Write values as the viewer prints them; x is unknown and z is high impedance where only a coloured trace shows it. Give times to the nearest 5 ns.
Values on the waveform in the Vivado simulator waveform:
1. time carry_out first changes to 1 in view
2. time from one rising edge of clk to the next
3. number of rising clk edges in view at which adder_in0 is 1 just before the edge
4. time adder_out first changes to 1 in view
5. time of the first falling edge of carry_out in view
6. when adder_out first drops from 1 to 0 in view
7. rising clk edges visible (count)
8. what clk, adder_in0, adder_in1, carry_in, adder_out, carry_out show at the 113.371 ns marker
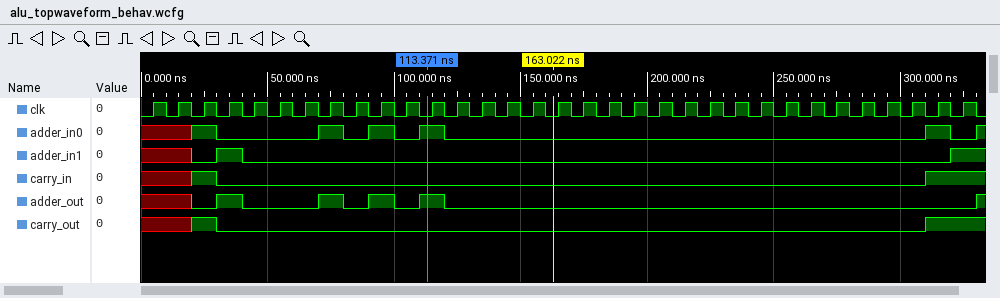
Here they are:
20 ns
10 ns
5
30 ns
30 ns
40 ns
33
clk=0, adder_in0=1, adder_in1=0, carry_in=0, adder_out=1, carry_out=0
